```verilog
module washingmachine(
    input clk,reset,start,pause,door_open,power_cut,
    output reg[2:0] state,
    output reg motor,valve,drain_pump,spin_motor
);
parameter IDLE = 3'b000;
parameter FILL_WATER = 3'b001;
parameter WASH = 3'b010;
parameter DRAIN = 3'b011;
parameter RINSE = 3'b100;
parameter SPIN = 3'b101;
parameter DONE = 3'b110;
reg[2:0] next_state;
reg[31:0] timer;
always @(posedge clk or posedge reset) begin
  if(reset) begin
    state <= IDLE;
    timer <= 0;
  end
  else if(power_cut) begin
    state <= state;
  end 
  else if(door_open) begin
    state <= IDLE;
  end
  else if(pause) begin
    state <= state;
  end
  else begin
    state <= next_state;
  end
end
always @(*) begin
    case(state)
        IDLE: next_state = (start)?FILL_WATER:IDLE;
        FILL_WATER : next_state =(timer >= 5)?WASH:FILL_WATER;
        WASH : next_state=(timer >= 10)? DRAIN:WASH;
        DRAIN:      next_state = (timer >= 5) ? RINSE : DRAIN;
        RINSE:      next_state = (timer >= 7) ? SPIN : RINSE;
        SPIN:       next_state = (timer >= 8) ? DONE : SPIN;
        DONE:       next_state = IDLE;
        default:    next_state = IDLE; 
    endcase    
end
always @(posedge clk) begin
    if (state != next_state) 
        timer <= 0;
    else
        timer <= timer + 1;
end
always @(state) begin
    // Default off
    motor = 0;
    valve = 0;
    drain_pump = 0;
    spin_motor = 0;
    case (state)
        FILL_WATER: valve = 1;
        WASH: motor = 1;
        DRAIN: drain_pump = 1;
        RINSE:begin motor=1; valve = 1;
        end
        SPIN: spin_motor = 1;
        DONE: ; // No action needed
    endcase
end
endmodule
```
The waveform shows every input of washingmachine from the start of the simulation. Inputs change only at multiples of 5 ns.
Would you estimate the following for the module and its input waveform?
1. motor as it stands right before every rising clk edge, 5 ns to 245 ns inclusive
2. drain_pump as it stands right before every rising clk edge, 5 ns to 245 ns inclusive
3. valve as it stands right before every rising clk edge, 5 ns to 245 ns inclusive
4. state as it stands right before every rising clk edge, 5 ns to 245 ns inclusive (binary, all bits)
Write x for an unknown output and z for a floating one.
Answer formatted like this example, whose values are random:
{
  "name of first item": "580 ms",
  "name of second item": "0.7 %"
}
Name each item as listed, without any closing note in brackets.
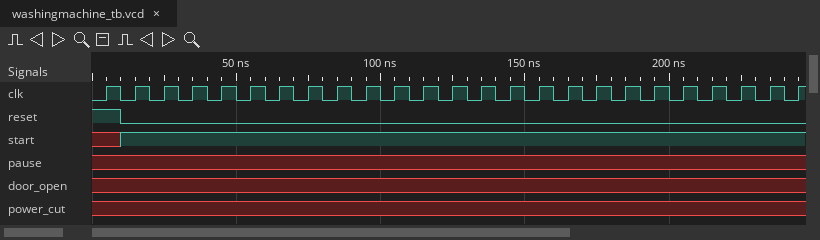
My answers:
{
  "motor as it stands right before every rising clk edge, 5 ns to 245 ns inclusive": "0 0 0 0 0 0 0 0 1 1 1 1 1 1 1 1 1 1 1 0 0 0 0 0 0",
  "drain_pump as it stands right before every rising clk edge, 5 ns to 245 ns inclusive": "0 0 0 0 0 0 0 0 0 0 0 0 0 0 0 0 0 0 0 1 1 1 1 1 1",
  "valve as it stands right before every rising clk edge, 5 ns to 245 ns inclusive": "0 0 1 1 1 1 1 1 0 0 0 0 0 0 0 0 0 0 0 0 0 0 0 0 0",
  "state as it stands right before every rising clk edge, 5 ns to 245 ns inclusive": "000, 000, 001, 001, 001, 001, 001, 001, 010, 010, 010, 010, 010, 010, 010, 010, 010, 010, 010, 011, 011, 011, 011, 011, 011"
}
